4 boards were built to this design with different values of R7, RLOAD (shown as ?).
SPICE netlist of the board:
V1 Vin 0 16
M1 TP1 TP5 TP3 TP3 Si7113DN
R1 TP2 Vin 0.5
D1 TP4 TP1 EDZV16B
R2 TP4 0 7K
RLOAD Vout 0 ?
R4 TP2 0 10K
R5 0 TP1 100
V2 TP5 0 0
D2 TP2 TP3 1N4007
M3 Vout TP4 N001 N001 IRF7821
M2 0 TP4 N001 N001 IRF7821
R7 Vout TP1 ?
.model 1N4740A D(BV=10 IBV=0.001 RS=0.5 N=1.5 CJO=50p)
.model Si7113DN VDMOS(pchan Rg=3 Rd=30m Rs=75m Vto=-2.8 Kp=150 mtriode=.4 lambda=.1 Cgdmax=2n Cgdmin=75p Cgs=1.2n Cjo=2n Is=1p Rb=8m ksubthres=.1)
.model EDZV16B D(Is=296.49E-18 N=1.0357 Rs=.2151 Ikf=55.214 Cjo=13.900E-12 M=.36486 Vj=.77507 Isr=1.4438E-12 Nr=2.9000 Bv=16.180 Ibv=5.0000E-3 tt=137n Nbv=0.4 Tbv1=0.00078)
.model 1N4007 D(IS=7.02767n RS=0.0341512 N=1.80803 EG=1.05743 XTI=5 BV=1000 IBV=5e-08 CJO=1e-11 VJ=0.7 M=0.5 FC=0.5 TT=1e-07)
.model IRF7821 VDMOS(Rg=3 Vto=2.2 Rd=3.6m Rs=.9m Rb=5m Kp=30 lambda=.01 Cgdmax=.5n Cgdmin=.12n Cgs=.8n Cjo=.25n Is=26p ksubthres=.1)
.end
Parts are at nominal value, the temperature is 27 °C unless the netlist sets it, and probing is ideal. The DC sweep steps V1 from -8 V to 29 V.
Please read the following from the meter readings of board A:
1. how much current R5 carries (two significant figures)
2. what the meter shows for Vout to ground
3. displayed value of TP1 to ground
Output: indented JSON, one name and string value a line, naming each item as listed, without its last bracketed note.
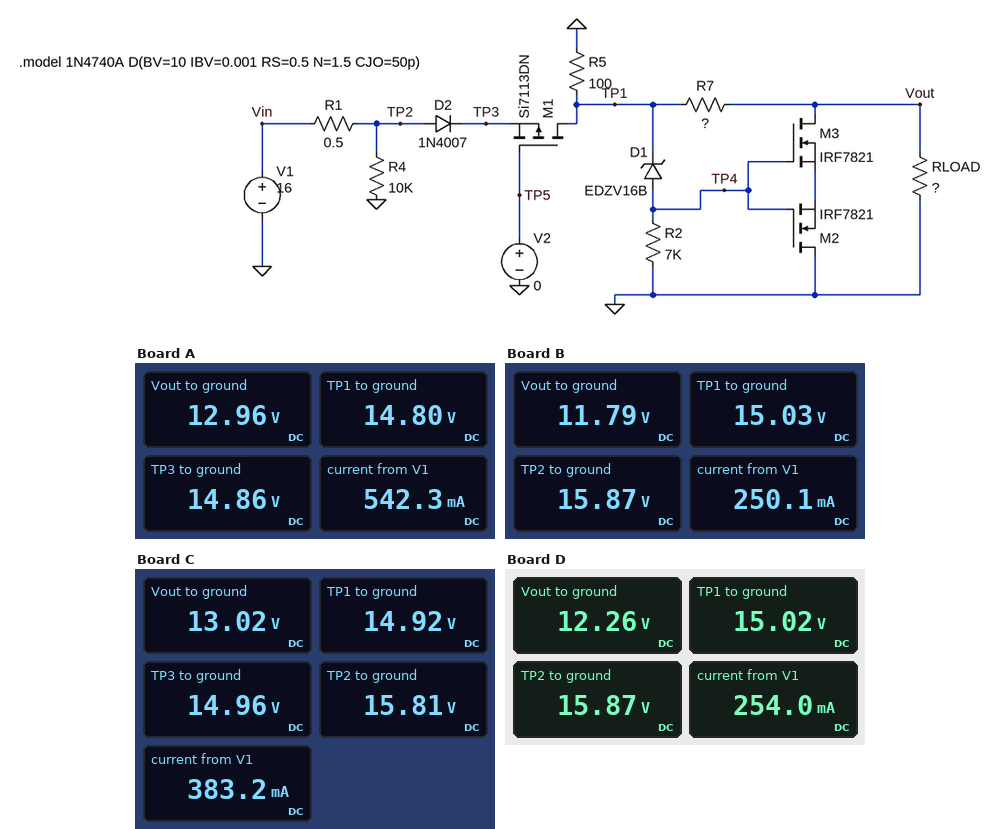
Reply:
{
  "how much current R5 carries": "150 mA",
  "what the meter shows for Vout to ground": "12.96 V",
  "displayed value of TP1 to ground": "14.80 V"
}
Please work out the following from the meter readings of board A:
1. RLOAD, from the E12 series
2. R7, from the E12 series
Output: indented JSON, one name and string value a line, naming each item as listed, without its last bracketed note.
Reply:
{
  "RLOAD, from the E12 series": "33 Ω",
  "R7, from the E12 series": "4.7 Ω"
}
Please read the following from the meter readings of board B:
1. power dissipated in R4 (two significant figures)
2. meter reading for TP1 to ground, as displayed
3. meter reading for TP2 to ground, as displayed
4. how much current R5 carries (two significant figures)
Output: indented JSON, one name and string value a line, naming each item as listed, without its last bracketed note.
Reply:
{
  "power dissipated in R4": "25 mW",
  "meter reading for TP1 to ground, as displayed": "15.03 V",
  "meter reading for TP2 to ground, as displayed": "15.87 V",
  "how much current R5 carries": "150 mA"
}
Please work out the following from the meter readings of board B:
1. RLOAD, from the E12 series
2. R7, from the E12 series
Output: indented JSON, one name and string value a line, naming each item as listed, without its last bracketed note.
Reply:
{
  "RLOAD, from the E12 series": "120 Ω",
  "R7, from the E12 series": "33 Ω"
}
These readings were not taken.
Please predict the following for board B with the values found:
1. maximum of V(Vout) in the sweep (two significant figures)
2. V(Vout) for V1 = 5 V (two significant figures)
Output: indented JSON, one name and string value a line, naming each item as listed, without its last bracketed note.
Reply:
{
  "maximum of V(Vout) in the sweep": "14 V",
  "V(Vout) for V1 = 5 V": "3.3 V"
}
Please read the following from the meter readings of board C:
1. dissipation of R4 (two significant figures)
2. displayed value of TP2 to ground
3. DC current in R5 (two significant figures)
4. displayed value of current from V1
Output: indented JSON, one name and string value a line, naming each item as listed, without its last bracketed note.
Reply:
{
  "dissipation of R4": "25 mW",
  "displayed value of TP2 to ground": "15.81 V",
  "DC current in R5": "150 mA",
  "displayed value of current from V1": "383.2 mA"
}
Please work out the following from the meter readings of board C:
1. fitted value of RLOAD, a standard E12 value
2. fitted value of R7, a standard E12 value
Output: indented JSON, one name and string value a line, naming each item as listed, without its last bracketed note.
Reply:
{
  "fitted value of RLOAD, a standard E12 value": "56 Ω",
  "fitted value of R7, a standard E12 value": "8.2 Ω"
}
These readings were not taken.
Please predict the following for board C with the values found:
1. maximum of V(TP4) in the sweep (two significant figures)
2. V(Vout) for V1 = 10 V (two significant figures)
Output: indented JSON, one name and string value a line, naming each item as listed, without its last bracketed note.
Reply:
{
  "maximum of V(TP4) in the sweep": "9.7 V",
  "V(Vout) for V1 = 10 V": "7.9 V"
}
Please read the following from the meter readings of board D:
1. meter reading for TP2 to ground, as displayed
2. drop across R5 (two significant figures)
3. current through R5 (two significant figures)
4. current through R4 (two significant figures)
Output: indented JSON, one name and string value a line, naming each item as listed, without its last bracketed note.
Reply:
{
  "meter reading for TP2 to ground, as displayed": "15.87 V",
  "drop across R5": "15 V",
  "current through R5": "150 mA",
  "current through R4": "1.6 mA"
}
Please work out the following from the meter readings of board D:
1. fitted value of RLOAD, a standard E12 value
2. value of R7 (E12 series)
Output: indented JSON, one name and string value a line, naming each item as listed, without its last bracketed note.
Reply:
{
  "fitted value of RLOAD, a standard E12 value": "120 Ω",
  "value of R7": "27 Ω"
}
